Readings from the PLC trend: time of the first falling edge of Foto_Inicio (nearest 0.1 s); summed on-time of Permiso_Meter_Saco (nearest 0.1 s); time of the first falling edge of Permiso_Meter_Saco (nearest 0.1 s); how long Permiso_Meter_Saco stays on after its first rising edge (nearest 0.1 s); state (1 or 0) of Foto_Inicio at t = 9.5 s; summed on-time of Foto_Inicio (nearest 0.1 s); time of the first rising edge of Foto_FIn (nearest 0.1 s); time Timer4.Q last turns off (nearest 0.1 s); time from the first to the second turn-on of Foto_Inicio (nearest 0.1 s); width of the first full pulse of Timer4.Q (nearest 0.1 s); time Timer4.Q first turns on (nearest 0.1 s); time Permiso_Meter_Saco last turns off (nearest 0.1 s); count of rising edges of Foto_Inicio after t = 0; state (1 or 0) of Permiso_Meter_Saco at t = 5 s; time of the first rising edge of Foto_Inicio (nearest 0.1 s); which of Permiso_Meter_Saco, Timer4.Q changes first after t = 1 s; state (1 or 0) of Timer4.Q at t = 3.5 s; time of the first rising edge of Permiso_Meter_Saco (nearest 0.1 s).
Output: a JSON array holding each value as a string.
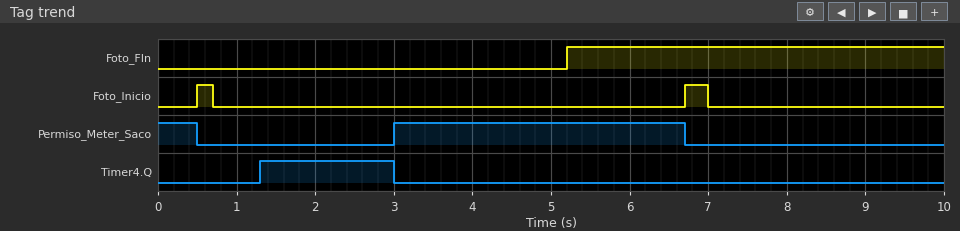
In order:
["0.7 s", "4.2 s", "0.5 s", "3.7 s", "0", "0.5 s", "5.2 s", "3.0 s", "6.2 s", "1.7 s", "1.3 s", "6.7 s", "2", "1", "0.5 s", "Timer4.Q", "0", "3.0 s"]
